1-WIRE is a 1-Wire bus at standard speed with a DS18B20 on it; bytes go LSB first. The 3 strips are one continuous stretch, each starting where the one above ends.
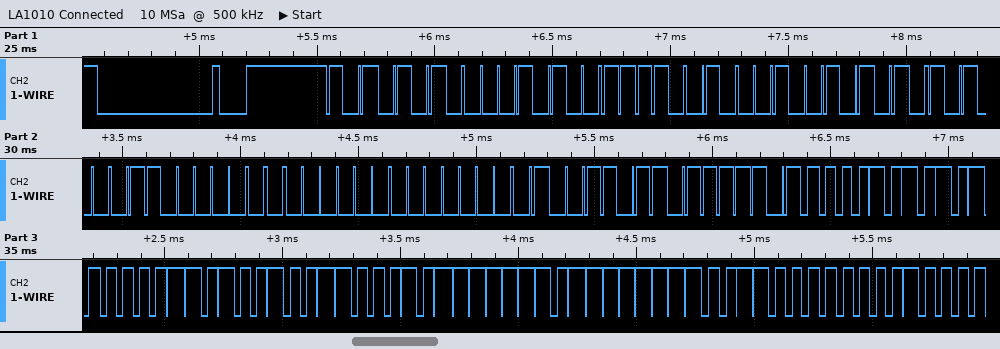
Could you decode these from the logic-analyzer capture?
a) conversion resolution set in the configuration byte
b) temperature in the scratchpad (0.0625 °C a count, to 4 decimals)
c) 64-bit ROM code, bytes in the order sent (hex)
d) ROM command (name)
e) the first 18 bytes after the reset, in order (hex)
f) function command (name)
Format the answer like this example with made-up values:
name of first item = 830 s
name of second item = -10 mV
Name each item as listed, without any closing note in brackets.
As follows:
conversion resolution set in the configuration byte = 12 bits
temperature in the scratchpad = 85.0000 °C
64-bit ROM code, bytes in the order sent = 28 4F A4 2A 06 00 00 D9
ROM command = Match ROM
the first 18 bytes after the reset, in order = 55 28 4F A4 2A 06 00 00 D9 BE 50 05 4B 46 7F FF 0C 10
function command = Read Scratchpad
